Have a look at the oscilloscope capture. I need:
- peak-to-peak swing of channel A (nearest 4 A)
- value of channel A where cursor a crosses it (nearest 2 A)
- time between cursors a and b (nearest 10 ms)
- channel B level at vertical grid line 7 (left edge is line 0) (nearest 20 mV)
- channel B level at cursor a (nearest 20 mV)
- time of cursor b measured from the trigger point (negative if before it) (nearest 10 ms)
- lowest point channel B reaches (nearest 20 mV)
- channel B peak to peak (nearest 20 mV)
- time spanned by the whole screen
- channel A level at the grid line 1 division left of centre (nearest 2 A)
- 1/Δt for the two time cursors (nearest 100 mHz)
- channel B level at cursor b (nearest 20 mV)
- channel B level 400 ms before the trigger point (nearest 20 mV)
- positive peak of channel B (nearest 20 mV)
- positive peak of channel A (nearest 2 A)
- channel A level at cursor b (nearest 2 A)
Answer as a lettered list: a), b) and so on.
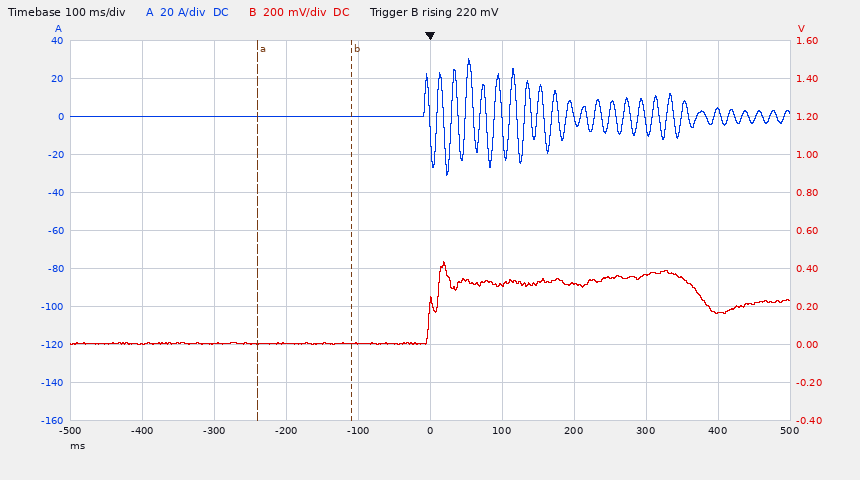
a) 60 A
b) 0 A
c) 130 ms
d) 320 mV
e) 0 mV
f) -110 ms
g) 0 mV
h) 440 mV
i) 1 s
j) 0 A
k) 7.7 Hz
l) 0 mV
m) 0 mV
n) 440 mV
o) 30 A
p) 0 A
